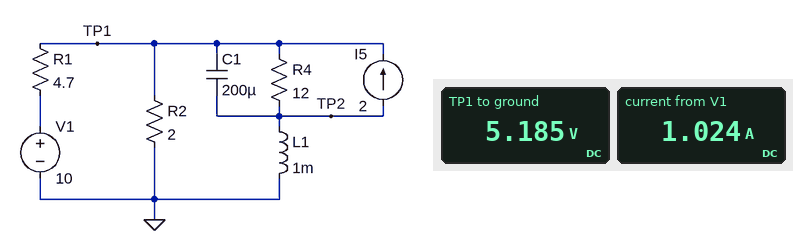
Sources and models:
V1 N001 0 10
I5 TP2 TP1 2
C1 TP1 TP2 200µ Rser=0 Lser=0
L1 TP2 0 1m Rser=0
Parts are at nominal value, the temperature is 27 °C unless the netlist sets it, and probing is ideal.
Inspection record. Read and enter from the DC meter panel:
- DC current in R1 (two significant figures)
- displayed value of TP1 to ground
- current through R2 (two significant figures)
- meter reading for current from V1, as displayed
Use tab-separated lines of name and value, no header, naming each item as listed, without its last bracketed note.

DC current in R1	1.0 A
displayed value of TP1 to ground	5.185 V
current through R2	2.6 A
meter reading for current from V1, as displayed	1.024 A
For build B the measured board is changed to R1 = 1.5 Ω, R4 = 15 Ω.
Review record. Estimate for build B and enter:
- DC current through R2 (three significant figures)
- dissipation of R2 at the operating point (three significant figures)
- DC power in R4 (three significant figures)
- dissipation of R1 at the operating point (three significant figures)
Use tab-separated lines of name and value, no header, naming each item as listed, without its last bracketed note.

DC current through R2	3.51 A
dissipation of R2 at the operating point	24.7 W
DC power in R4	3.29 W
dissipation of R1 at the operating point	5.89 W
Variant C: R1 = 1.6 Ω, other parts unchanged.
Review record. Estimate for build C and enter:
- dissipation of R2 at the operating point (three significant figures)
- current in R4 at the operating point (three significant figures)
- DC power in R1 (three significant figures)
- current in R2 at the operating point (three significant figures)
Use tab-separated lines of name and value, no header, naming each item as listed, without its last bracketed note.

dissipation of R2 at the operating point	23.3 W
current in R4 at the operating point	569 mA
DC power in R1	6.29 W
current in R2 at the operating point	3.41 A
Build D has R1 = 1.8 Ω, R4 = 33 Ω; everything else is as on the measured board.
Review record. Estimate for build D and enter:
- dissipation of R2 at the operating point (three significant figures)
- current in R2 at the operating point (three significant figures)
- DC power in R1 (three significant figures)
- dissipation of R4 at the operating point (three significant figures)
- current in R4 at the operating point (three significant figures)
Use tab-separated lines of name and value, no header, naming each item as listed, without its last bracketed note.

dissipation of R2 at the operating point	24.2 W
current in R2 at the operating point	3.48 A
DC power in R1	5.14 W
dissipation of R4 at the operating point	1.47 W
current in R4 at the operating point	211 mA
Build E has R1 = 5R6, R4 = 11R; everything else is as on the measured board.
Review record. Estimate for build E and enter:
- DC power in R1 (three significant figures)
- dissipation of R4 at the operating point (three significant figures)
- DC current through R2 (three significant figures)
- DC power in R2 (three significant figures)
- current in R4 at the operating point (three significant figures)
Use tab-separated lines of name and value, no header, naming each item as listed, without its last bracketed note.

DC power in R1	4.61 W
dissipation of R4 at the operating point	2.20 W
DC current through R2	2.46 A
DC power in R2	12.1 W
current in R4 at the operating point	447 mA
